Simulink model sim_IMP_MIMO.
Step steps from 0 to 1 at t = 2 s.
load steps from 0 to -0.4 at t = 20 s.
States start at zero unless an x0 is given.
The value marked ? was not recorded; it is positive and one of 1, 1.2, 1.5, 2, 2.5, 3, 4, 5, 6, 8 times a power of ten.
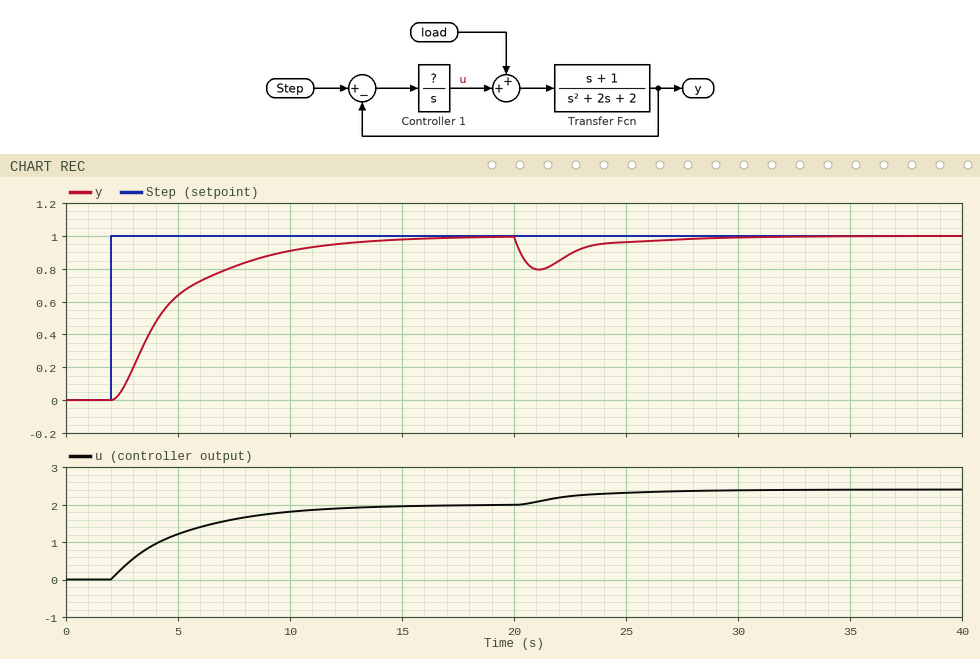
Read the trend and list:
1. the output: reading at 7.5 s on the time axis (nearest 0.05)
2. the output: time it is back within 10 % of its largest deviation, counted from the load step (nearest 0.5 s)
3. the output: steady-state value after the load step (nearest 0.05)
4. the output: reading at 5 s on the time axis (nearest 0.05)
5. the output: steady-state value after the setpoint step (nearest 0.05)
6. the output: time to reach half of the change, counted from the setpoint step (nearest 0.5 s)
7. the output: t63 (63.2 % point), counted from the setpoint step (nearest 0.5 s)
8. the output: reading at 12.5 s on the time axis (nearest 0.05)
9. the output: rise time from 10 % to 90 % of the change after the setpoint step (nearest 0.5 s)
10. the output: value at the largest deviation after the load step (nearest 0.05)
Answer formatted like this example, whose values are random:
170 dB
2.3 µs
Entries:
0.80
7.5 s
1.00
0.65
1.00
2.0 s
3.0 s
0.95
7.0 s
0.80
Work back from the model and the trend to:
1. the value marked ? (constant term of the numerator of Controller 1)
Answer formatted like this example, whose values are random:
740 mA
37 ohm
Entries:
0.6
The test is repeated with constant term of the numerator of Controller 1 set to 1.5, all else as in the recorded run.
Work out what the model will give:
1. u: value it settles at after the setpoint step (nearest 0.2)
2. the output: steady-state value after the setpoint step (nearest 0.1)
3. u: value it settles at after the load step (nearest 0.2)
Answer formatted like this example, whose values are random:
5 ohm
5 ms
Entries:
2.0
1.0
2.4
